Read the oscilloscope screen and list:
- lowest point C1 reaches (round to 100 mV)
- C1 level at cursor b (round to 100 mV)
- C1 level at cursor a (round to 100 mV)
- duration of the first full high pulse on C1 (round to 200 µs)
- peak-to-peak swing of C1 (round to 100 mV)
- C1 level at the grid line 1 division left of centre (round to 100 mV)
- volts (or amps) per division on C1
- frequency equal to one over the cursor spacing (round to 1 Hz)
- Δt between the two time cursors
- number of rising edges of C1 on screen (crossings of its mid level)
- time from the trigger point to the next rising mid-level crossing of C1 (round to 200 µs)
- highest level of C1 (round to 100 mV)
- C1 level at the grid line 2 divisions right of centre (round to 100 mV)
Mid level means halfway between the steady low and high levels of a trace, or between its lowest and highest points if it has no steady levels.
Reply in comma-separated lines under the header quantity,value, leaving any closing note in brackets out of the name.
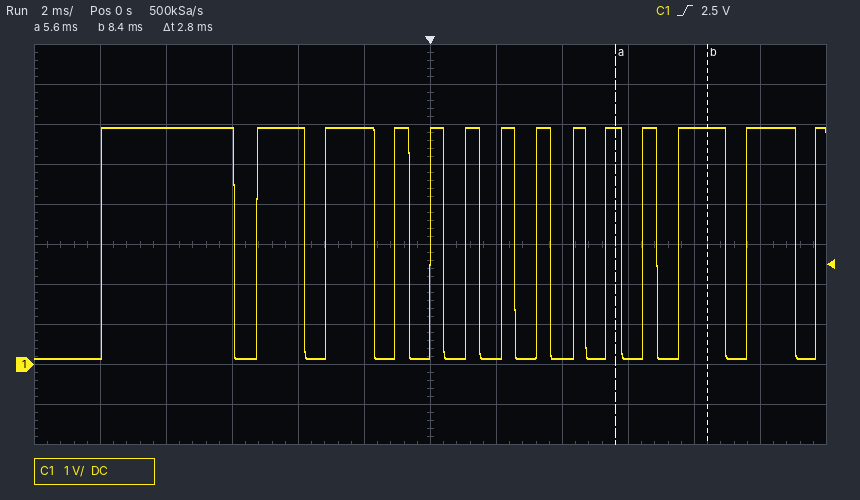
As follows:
quantity,value
lowest point C1 reaches,100 mV
C1 level at cursor b,5.9 V
C1 level at cursor a,5.9 V
duration of the first full high pulse on C1,4.0 ms
peak-to-peak swing of C1,5.8 V
C1 level at the grid line 1 division left of centre,5.9 V
volts (or amps) per division on C1,1 V
frequency equal to one over the cursor spacing,357 Hz
Δt between the two time cursors,2.8 ms
number of rising edges of C1 on screen,14
time from the trigger point to the next rising mid-level crossing of C1,1.0 ms
highest level of C1,5.9 V
C1 level at the grid line 2 divisions right of centre,100 mV
